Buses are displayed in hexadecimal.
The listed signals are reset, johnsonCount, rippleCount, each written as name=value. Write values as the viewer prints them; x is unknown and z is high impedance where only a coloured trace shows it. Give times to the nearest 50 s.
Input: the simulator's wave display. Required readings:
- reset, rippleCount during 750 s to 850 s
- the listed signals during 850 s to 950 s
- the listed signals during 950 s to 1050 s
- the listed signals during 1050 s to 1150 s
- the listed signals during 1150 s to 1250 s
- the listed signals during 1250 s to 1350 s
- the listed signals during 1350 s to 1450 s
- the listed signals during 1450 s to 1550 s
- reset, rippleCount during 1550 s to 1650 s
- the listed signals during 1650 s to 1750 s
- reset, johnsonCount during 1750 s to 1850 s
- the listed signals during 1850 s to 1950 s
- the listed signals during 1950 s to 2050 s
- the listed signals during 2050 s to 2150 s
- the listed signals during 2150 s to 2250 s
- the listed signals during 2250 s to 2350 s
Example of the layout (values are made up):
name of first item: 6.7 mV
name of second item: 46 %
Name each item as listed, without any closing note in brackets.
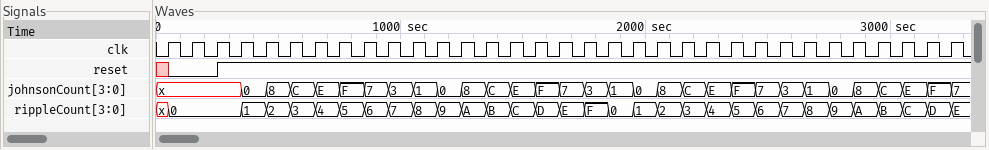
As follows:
reset, rippleCount during 750 s to 850 s: reset=1, rippleCount=5
the listed signals during 850 s to 950 s: reset=1, johnsonCount=7, rippleCount=6
the listed signals during 950 s to 1050 s: reset=1, johnsonCount=3, rippleCount=7
the listed signals during 1050 s to 1150 s: reset=1, johnsonCount=1, rippleCount=8
the listed signals during 1150 s to 1250 s: reset=1, johnsonCount=0, rippleCount=9
the listed signals during 1250 s to 1350 s: reset=1, johnsonCount=8, rippleCount=A
the listed signals during 1350 s to 1450 s: reset=1, johnsonCount=C, rippleCount=B
the listed signals during 1450 s to 1550 s: reset=1, johnsonCount=E, rippleCount=C
reset, rippleCount during 1550 s to 1650 s: reset=1, rippleCount=D
the listed signals during 1650 s to 1750 s: reset=1, johnsonCount=7, rippleCount=E
reset, johnsonCount during 1750 s to 1850 s: reset=1, johnsonCount=3
the listed signals during 1850 s to 1950 s: reset=1, johnsonCount=1, rippleCount=0
the listed signals during 1950 s to 2050 s: reset=1, johnsonCount=0, rippleCount=1
the listed signals during 2050 s to 2150 s: reset=1, johnsonCount=8, rippleCount=2
the listed signals during 2150 s to 2250 s: reset=1, johnsonCount=C, rippleCount=3
the listed signals during 2250 s to 2350 s: reset=1, johnsonCount=E, rippleCount=4
